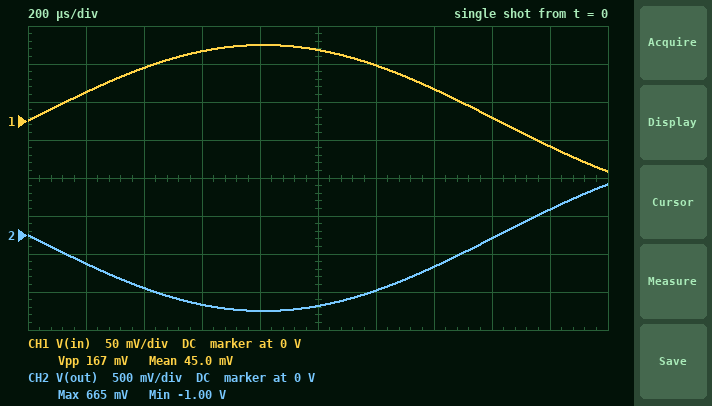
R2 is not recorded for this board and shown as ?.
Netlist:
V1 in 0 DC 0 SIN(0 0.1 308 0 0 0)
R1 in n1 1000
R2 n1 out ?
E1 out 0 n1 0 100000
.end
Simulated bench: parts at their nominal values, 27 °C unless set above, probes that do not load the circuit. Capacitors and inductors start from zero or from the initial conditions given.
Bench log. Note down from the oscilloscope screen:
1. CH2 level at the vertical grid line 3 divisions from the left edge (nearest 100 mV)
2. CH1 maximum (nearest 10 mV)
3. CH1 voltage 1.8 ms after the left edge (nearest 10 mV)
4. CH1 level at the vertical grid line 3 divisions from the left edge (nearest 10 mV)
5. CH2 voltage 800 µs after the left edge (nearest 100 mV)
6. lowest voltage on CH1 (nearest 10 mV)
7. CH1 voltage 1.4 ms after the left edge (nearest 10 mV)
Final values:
-900 mV
100 mV
-30 mV
90 mV
-1.0 V
-70 mV
40 mV
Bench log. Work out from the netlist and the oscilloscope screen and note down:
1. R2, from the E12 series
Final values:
10 kΩ
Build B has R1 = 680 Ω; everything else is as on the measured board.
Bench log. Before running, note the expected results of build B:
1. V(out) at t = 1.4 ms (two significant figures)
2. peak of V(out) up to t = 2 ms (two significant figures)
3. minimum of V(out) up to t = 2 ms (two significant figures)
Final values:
-620 mV
980 mV
-1.5 V
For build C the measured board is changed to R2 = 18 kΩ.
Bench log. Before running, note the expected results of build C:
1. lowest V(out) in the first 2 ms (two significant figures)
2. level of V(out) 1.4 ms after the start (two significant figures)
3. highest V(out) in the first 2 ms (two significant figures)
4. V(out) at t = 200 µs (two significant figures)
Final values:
-1.8 V
-750 mV
1.2 V
-680 mV
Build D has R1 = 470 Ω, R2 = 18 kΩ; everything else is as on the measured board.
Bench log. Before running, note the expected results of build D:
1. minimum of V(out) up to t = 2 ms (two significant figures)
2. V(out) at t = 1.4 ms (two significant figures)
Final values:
-3.8 V
-1.6 V
